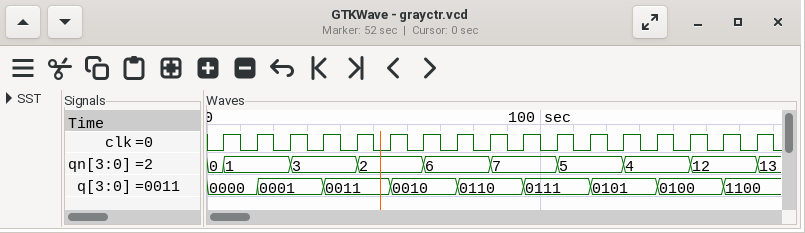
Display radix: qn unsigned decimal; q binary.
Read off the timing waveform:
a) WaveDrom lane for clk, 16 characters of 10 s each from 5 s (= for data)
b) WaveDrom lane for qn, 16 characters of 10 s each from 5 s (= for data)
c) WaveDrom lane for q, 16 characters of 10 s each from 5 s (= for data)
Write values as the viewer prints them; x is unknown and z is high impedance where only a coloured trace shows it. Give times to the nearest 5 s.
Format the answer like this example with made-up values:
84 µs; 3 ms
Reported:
{name: 'clk', wave: 'p...............'}; {name: 'qn', wave: '=.=.=.=.=.=.=.=.', data: '1 3 2 6 7 5 4 12'}; {name: 'q', wave: '==.=.=.=.=.=.=.=', data: '0000 0001 0011 0010 0110 0111 0101 0100 1100'}
